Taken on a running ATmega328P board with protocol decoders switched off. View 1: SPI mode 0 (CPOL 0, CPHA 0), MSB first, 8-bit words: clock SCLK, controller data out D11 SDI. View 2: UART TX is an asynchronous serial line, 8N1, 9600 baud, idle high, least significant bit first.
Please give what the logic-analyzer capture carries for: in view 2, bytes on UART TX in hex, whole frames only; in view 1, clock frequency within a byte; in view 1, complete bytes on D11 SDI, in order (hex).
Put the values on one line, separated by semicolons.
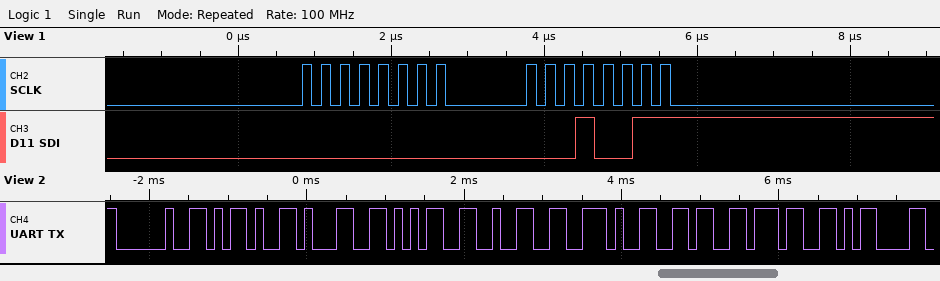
20 2D 31 35 32 2E 36 37 0D; 4 MHz; 00 13
